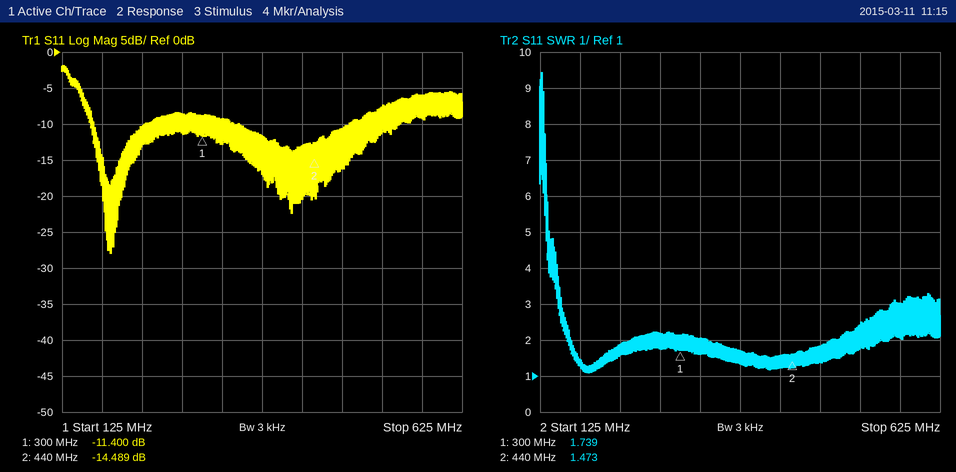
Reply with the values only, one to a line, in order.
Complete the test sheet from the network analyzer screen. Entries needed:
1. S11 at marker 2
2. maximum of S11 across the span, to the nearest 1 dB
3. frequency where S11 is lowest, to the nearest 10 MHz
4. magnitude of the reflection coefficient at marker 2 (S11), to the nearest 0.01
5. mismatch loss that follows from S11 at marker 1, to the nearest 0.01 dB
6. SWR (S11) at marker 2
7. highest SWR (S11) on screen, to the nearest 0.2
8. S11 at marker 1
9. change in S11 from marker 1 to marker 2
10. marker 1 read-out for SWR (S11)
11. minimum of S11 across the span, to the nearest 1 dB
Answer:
-14.489 dB
-2 dB
190 MHz
0.19
0.33 dB
1.473
9.4
-11.400 dB
-3.089 dB
1.739
-28 dB
